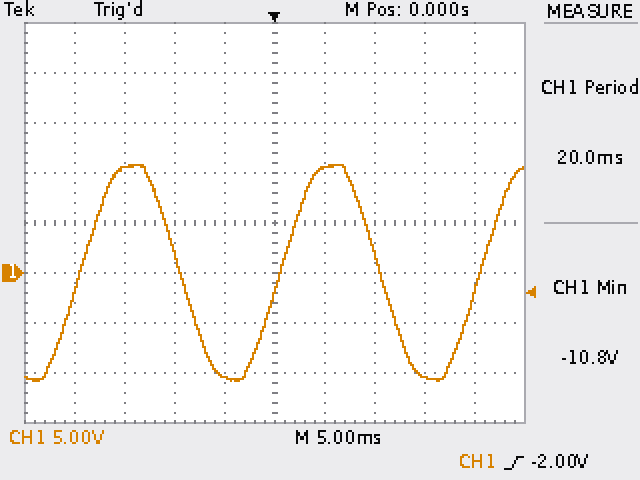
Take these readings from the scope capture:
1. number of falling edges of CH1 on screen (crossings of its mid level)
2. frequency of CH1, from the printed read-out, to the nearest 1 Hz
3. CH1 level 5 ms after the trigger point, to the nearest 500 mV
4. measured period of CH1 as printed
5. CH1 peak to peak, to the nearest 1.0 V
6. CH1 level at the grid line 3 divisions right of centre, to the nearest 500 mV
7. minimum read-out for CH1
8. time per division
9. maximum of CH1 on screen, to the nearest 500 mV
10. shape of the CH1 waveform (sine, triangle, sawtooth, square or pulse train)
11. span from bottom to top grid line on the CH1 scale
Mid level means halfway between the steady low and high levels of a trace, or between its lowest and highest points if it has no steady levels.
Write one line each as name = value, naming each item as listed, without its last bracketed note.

number of falling edges of CH1 on screen = 2
frequency of CH1, from the printed read-out, to the nearest 1 Hz = 50 Hz
CH1 level 5 ms after the trigger point, to the nearest 500 mV = 10.5 V
measured period of CH1 as printed = 20.0 ms
CH1 peak to peak, to the nearest 1.0 V = 22.0 V
CH1 level at the grid line 3 divisions right of centre, to the nearest 500 mV = -10.5 V
minimum read-out for CH1 = -10.8 V
time per division = 5 ms
maximum of CH1 on screen, to the nearest 500 mV = 11.0 V
shape of the CH1 waveform = sine
span from bottom to top grid line on the CH1 scale = 40 V
